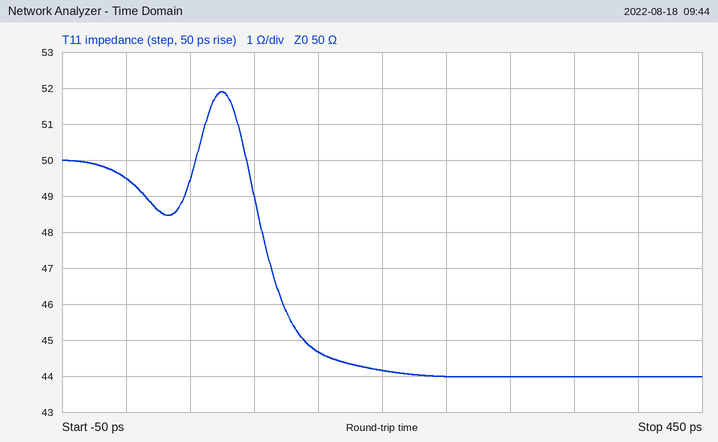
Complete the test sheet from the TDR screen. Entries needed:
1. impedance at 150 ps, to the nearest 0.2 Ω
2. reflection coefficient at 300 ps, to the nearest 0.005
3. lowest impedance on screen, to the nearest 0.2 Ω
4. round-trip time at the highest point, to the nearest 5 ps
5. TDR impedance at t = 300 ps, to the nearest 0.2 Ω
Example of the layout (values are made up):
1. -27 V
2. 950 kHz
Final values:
1. 44.6 Ω
2. -0.065
3. 44.0 Ω
4. 75 ps
5. 44.0 Ω
